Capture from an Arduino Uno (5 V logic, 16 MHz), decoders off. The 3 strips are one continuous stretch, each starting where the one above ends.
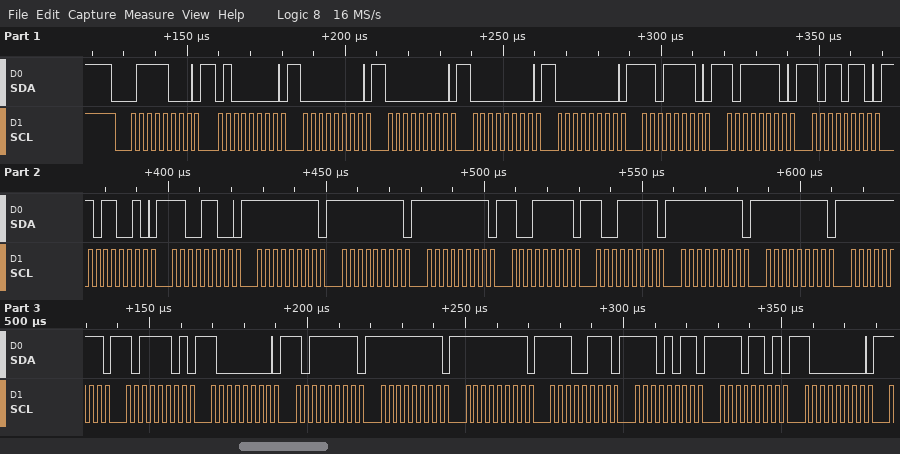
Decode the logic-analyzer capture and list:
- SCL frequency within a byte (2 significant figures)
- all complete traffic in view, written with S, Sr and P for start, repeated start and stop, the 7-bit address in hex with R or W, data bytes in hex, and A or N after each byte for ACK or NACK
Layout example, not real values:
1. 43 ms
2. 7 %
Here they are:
1. 400 kHz
2. S 3CW A 40 A 00 A 00 A 00 A 00 A DE A BE A B6 A B2 A CC A FF A FF A FF A 9F A 9F A FF A FF A FF A BD A 80 A BF A FF A FF A E7 A EB A ED A 80 A
